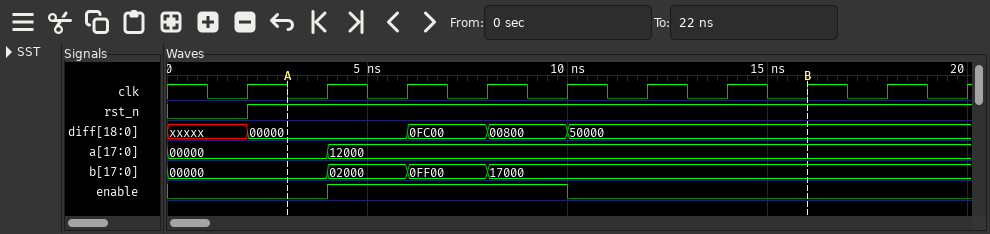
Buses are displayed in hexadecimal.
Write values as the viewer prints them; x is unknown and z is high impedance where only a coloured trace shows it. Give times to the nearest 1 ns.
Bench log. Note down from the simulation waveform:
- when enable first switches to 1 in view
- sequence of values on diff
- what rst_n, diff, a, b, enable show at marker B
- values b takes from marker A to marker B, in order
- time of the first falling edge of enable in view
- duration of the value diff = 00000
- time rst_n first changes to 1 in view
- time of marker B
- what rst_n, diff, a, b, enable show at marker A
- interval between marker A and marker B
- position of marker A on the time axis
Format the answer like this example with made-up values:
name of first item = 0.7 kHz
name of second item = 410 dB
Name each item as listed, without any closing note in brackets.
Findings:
when enable first switches to 1 in view = 4 ns
sequence of values on diff = xxxxx, 00000, 0FC00, 00800, 50000
what rst_n, diff, a, b, enable show at marker B = rst_n=1, diff=50000, a=12000, b=17000, enable=0
values b takes from marker A to marker B, in order = 00000, 02000, 0FF00, 17000
time of the first falling edge of enable in view = 10 ns
duration of the value diff = 00000 = 4 ns
time rst_n first changes to 1 in view = 2 ns
time of marker B = 16 ns
what rst_n, diff, a, b, enable show at marker A = rst_n=1, diff=00000, a=00000, b=00000, enable=0
interval between marker A and marker B = 13 ns
position of marker A on the time axis = 3 ns
